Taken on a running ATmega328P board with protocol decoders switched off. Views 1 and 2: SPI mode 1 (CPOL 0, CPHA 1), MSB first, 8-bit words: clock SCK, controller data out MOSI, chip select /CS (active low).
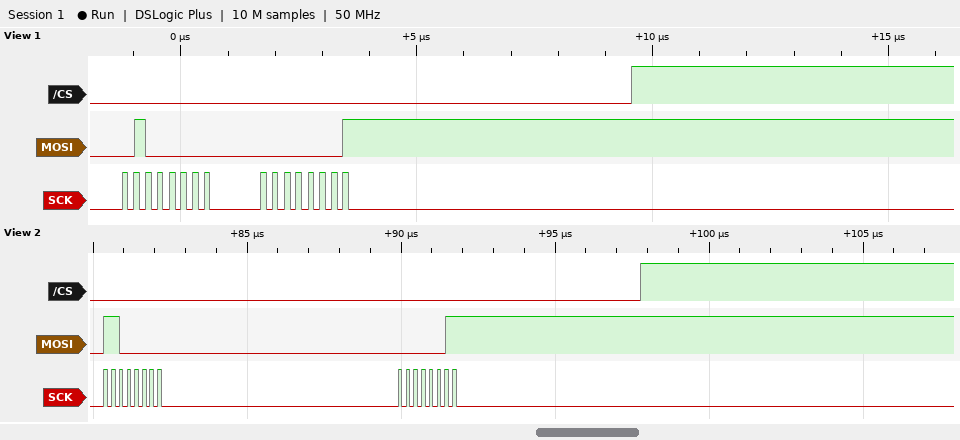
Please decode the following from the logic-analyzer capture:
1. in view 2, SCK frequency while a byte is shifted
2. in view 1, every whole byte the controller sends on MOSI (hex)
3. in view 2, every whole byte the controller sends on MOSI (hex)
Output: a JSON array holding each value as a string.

["4 MHz", "40 01", "C0 03"]
